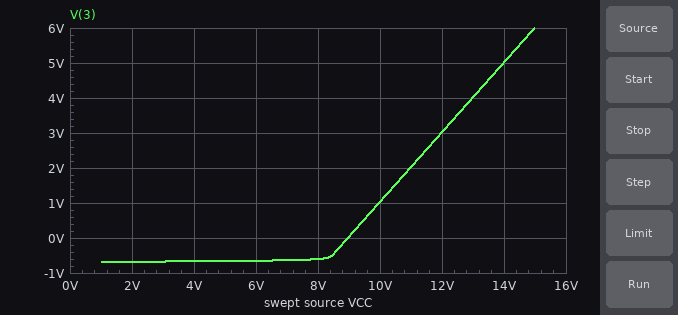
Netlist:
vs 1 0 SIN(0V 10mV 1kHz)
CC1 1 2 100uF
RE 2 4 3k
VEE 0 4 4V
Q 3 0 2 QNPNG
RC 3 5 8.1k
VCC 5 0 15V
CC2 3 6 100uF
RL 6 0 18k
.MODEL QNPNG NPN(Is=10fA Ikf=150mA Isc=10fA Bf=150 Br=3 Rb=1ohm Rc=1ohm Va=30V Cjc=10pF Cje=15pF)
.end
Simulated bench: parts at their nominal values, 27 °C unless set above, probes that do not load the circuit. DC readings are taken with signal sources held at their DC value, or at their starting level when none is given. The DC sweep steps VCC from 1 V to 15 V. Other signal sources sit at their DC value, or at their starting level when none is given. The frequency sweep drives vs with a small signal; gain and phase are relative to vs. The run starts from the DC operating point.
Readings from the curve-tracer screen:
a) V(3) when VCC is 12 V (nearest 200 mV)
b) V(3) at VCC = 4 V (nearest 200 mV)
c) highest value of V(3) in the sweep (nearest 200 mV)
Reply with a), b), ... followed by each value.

a) 3.0 V
b) -600 mV
c) 6.0 V
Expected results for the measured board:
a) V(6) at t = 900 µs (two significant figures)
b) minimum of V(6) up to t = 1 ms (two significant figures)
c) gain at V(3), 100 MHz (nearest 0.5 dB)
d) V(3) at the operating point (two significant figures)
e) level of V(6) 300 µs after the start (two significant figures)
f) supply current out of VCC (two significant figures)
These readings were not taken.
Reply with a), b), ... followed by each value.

a) -1.2 V
b) -2.4 V
c) 22.5 dB
d) 6.0 V
e) 1.6 V
f) 1.1 mA
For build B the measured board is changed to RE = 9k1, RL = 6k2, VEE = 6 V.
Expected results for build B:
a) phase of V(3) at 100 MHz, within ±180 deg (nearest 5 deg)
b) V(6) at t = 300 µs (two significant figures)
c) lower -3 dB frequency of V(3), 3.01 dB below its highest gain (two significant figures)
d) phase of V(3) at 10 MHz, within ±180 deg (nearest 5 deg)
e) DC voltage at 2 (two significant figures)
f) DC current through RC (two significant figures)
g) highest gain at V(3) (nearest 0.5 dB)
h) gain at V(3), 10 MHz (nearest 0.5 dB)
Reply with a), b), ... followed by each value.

a) -85 deg
b) 590 mV
c) 35 Hz
d) -40 deg
e) -630 mV
f) 590 µA
g) 37.5 dB
h) 35.0 dB
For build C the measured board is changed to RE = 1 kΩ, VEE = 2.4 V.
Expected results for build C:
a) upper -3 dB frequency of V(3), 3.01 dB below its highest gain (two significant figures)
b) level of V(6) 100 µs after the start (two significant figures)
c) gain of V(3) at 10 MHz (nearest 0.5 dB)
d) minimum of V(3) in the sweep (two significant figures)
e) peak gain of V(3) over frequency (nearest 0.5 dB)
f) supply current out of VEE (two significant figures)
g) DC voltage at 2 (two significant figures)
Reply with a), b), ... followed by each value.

a) 4.7 MHz
b) 1.5 V
c) 41.5 dB
d) -690 mV
e) 49.0 dB
f) 1.7 mA
g) -670 mV
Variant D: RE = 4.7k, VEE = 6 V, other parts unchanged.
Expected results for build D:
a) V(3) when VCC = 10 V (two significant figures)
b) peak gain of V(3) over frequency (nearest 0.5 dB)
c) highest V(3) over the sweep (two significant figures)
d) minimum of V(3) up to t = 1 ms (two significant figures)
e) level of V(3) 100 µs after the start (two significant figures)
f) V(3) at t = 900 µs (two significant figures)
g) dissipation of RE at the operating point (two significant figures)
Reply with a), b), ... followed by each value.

a) 850 mV
b) 46.5 dB
c) 5.8 V
d) 3.4 V
e) 6.9 V
f) 4.6 V
g) 6.1 mW
